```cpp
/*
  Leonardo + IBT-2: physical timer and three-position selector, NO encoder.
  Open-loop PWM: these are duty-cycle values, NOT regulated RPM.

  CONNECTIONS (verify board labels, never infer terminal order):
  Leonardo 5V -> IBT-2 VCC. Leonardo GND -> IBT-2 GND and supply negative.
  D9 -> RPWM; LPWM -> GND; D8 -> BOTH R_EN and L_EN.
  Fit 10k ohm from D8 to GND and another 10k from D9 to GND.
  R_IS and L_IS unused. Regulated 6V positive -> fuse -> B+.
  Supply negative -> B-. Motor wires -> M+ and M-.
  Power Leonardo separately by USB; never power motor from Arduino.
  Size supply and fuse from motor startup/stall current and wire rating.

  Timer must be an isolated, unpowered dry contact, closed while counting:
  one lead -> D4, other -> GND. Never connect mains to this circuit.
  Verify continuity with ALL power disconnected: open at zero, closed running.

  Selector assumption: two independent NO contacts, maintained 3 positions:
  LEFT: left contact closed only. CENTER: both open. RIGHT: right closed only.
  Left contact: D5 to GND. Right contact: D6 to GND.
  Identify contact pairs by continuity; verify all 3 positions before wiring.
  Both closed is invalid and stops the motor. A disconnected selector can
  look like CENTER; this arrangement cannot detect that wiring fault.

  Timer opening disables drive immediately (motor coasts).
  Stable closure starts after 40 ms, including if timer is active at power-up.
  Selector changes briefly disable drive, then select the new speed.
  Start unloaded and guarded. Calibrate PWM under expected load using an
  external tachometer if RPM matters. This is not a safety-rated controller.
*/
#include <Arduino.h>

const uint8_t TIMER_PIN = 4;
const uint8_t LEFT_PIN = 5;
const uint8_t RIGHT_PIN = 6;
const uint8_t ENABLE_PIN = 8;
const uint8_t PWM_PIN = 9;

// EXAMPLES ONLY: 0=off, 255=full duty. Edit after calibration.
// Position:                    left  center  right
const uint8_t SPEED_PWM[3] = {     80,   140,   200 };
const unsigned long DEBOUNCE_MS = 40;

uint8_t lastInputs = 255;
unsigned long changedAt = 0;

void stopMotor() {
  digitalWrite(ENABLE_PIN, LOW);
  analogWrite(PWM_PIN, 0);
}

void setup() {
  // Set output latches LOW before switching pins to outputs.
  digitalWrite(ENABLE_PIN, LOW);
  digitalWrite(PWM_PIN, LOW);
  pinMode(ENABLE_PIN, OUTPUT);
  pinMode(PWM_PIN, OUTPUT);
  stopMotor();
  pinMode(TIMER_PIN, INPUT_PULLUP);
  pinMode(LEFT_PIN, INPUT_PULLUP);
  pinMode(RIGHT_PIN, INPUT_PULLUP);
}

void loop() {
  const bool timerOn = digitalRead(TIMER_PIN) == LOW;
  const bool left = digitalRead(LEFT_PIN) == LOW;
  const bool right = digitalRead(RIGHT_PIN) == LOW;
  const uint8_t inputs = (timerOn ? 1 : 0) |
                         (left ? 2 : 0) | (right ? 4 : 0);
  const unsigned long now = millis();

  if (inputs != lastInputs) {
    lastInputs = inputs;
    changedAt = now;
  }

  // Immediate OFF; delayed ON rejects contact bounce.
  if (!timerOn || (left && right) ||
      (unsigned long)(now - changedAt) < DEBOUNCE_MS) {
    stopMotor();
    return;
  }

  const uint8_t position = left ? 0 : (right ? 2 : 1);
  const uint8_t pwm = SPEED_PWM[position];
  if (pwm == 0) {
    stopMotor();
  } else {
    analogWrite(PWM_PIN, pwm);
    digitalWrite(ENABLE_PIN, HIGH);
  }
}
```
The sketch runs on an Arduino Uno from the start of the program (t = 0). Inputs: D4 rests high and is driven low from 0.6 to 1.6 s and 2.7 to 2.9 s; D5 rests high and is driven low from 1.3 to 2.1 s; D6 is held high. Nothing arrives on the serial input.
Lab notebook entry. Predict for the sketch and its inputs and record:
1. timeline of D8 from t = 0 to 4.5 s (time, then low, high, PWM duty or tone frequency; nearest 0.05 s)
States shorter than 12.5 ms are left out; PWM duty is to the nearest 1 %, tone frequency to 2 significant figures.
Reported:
0 s low; 0.65 s high; 1.3 s low; 1.35 s high; 1.6 s low; 2.75 s high; 2.9 s low
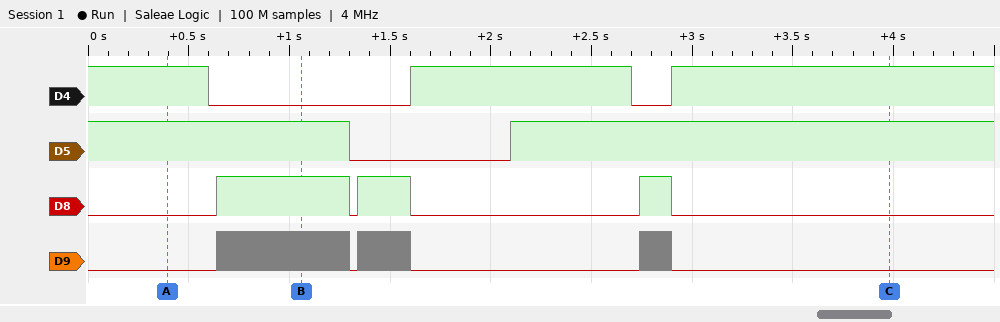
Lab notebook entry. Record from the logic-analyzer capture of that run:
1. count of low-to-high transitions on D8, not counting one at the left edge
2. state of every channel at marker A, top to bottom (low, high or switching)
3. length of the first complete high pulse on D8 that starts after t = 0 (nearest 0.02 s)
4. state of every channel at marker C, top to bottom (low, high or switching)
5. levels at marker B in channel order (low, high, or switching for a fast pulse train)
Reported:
3
D4 high, D5 high, D8 low, D9 low
0.66 s
D4 high, D5 high, D8 low, D9 low
D4 low, D5 high, D8 high, D9 switching
